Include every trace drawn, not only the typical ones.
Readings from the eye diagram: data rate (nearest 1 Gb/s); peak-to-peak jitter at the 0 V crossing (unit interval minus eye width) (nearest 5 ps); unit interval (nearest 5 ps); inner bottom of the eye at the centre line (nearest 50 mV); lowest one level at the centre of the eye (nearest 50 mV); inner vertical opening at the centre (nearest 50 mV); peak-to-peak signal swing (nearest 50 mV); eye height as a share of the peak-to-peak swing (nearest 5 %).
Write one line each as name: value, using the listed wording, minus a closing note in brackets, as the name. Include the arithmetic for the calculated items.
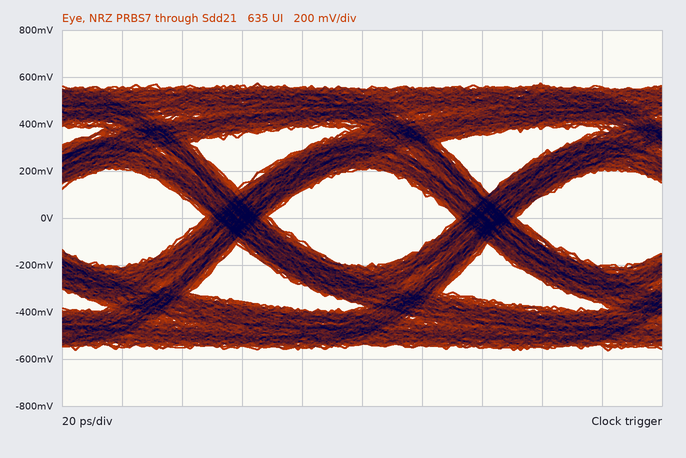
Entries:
data rate: 12 Gb/s
peak-to-peak jitter at the 0 V crossing (unit interval minus eye width): 20 ps
unit interval: 85 ps
inner bottom of the eye at the centre line: -200 mV
lowest one level at the centre of the eye: 200 mV
inner vertical opening at the centre: 400 mV
peak-to-peak signal swing: 1.15 V
eye height as a share of the peak-to-peak swing: 400 mV / 1.15 V ≈ 35 %
